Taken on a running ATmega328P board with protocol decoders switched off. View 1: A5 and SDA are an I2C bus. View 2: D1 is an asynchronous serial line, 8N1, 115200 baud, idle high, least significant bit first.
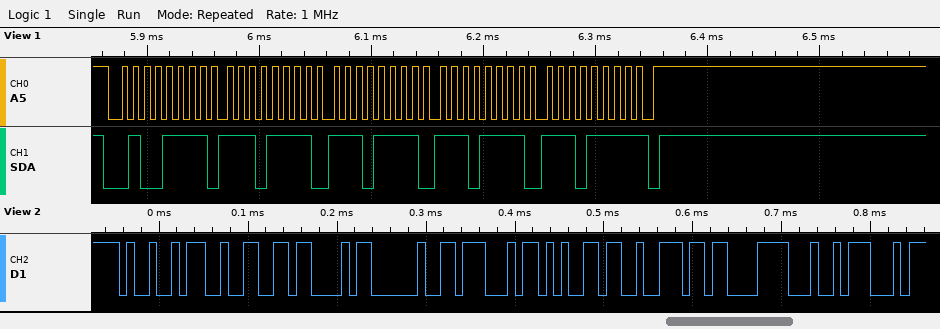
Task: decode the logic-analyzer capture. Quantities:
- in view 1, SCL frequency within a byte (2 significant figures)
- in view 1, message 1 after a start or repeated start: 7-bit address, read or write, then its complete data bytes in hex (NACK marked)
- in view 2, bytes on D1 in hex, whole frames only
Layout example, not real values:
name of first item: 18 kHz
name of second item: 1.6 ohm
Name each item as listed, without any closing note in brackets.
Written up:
in view 1, SCL frequency within a byte: 100 kHz
in view 1, message 1 after a start or repeated start: 7-bit address, read or write, then its complete data bytes in hex: 0x27 read: EF EF EF EF NACK
in view 2, bytes on D1 in hex, whole frames only: 49 32 43 20 47 65 72 C3 A4
